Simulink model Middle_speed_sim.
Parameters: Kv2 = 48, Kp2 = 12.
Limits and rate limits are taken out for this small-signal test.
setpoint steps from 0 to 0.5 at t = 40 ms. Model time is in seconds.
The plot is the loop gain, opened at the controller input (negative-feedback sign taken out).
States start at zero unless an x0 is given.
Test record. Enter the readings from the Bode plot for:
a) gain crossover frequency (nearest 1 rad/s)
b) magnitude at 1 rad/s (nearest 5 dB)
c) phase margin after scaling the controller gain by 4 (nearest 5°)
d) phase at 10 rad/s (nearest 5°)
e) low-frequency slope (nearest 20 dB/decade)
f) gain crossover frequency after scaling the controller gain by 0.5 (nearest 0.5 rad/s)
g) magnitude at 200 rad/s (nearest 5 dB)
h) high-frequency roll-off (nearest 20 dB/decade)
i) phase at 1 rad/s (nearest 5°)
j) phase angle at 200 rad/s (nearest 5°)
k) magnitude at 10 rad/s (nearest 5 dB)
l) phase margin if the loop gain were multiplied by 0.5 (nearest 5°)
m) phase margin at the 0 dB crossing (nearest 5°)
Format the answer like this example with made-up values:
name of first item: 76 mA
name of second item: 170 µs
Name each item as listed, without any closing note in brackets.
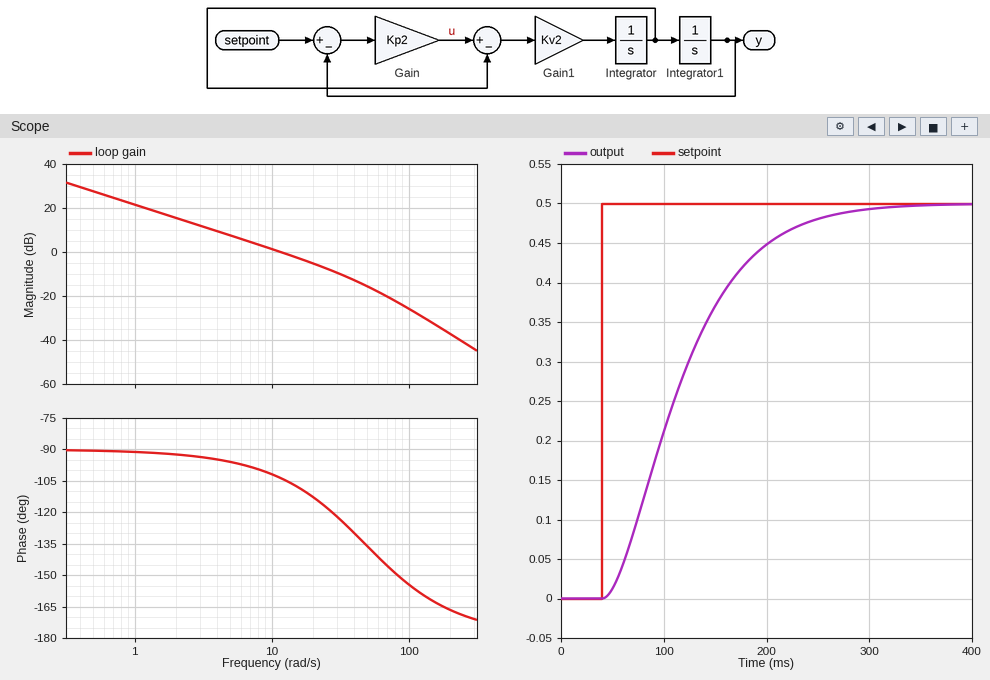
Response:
gain crossover frequency: 12 rad/s
magnitude at 1 rad/s: 20 dB
phase margin after scaling the controller gain by 4: 50°
phase at 10 rad/s: -100°
low-frequency slope: -20 dB/decade
gain crossover frequency after scaling the controller gain by 0.5: 6.0 rad/s
magnitude at 200 rad/s: -35 dB
high-frequency roll-off: -40 dB/decade
phase at 1 rad/s: -90°
phase angle at 200 rad/s: -165°
magnitude at 10 rad/s: 0 dB
phase margin if the loop gain were multiplied by 0.5: 85°
phase margin at the 0 dB crossing: 75°
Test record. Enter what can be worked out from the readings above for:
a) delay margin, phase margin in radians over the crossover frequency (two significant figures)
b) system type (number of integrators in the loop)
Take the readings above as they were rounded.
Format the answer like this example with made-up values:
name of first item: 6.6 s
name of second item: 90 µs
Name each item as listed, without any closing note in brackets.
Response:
delay margin, phase margin in radians over the crossover frequency: 0.11 s
system type: 1
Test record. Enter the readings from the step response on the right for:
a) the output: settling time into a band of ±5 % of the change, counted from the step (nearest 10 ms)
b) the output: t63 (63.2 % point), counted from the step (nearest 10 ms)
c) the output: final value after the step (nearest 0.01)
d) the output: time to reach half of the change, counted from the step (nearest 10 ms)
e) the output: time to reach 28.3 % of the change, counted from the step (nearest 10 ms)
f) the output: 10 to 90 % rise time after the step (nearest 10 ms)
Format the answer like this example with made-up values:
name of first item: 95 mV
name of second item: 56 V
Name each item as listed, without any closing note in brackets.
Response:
the output: settling time into a band of ±5 % of the change, counted from the step: 200 ms
the output: t63 (63.2 % point), counted from the step: 90 ms
the output: final value after the step: 0.50
the output: time to reach half of the change, counted from the step: 70 ms
the output: time to reach 28.3 % of the change, counted from the step: 40 ms
the output: 10 to 90 % rise time after the step: 140 ms
